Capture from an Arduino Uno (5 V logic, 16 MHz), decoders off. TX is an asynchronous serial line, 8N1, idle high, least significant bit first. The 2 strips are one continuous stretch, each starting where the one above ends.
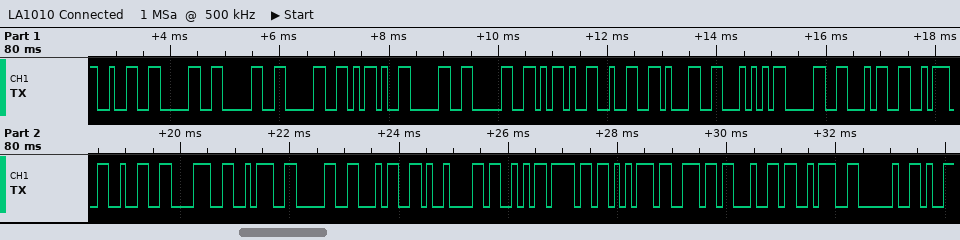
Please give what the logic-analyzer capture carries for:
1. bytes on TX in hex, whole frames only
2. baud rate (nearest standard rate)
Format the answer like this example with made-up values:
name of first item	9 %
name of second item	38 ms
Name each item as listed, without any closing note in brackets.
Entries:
bytes on TX in hex, whole frames only	0x32 0x30 0x30 0x30 0x2D 0x30 0x30 0x2D 0x32 0x31 0x54 0x30 0x34 0x3A 0x32 0x38 0x3A 0x30 0x34 0x09 0x53 0x6F 0x75 0x6E 0x64 0x3A 0x20
baud rate	9600 baud
